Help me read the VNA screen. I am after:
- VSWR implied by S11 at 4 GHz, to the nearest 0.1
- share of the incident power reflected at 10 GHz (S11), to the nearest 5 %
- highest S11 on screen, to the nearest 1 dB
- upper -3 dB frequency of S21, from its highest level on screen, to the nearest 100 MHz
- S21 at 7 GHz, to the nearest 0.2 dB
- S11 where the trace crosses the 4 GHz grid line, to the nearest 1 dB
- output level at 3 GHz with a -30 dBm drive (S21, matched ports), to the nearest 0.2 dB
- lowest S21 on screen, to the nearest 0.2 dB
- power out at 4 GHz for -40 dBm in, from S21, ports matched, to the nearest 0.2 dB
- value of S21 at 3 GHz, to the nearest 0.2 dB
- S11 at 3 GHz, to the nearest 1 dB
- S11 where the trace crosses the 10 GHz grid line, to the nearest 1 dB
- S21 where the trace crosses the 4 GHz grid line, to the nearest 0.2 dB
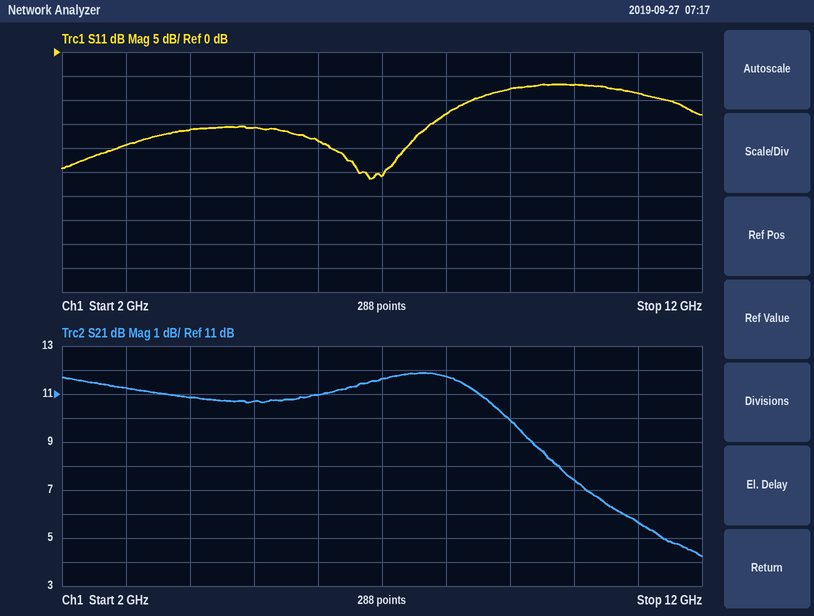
1.4
20 %
-7 dB
9.4 GHz
11.6 dB
-16 dB
-18.8 dBm
4.2 dB
-29.2 dBm
11.2 dB
-19 dB
-7 dB
10.8 dB
